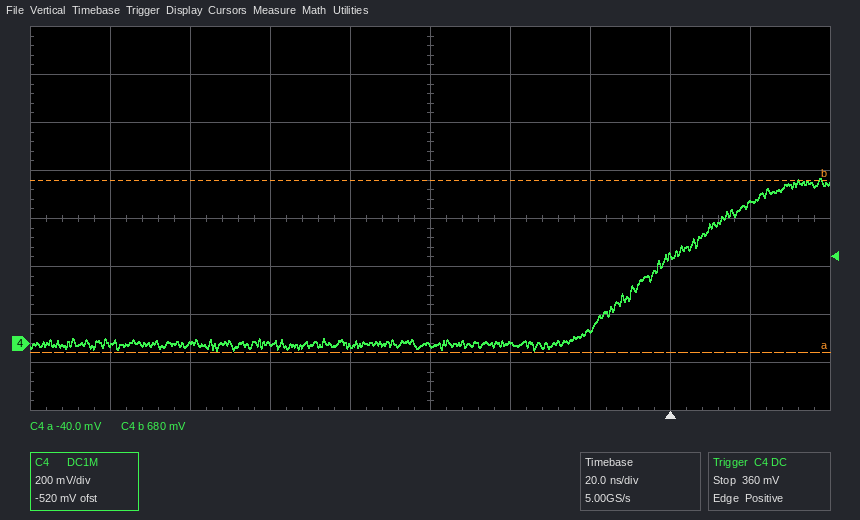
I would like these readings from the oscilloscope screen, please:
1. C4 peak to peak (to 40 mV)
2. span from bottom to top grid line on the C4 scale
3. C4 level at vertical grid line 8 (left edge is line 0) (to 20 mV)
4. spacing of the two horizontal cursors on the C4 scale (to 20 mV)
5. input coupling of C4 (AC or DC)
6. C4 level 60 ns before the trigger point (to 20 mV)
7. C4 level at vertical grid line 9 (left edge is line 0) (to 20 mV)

720 mV
1.6 V
360 mV
720 mV
DC
0 mV
580 mV
